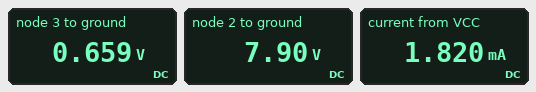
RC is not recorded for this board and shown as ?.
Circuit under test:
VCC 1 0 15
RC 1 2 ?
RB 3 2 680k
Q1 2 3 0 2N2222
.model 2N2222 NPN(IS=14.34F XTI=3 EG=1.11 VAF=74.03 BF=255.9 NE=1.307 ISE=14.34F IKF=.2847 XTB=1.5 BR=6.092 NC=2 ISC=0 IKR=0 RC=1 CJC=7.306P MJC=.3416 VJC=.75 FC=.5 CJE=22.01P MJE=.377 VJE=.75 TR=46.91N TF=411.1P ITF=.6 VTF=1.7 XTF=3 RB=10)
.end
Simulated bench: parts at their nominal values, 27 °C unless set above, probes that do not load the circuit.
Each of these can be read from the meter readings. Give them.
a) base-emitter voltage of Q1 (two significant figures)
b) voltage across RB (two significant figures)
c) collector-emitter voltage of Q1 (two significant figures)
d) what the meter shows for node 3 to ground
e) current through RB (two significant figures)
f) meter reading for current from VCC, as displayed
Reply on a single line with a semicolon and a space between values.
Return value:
660 mV; 7.2 V; 7.9 V; 0.659 V; 11 µA; 1.820 mA
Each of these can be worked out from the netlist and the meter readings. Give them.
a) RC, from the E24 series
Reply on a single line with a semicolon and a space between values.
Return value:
3.9 kΩ
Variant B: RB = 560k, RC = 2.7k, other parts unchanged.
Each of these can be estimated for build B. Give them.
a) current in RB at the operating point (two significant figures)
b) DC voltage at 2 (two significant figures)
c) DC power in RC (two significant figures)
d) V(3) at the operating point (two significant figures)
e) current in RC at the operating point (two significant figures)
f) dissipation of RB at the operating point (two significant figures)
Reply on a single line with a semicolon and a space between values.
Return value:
14 µA; 8.4 V; 16 mW; 670 mV; 2.4 mA; 110 µW
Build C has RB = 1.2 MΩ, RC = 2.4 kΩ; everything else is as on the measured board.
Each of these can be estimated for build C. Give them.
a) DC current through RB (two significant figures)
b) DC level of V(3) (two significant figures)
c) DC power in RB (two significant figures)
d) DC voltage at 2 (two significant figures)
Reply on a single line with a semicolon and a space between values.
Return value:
8.9 µA; 650 mV; 94 µW; 11 V
